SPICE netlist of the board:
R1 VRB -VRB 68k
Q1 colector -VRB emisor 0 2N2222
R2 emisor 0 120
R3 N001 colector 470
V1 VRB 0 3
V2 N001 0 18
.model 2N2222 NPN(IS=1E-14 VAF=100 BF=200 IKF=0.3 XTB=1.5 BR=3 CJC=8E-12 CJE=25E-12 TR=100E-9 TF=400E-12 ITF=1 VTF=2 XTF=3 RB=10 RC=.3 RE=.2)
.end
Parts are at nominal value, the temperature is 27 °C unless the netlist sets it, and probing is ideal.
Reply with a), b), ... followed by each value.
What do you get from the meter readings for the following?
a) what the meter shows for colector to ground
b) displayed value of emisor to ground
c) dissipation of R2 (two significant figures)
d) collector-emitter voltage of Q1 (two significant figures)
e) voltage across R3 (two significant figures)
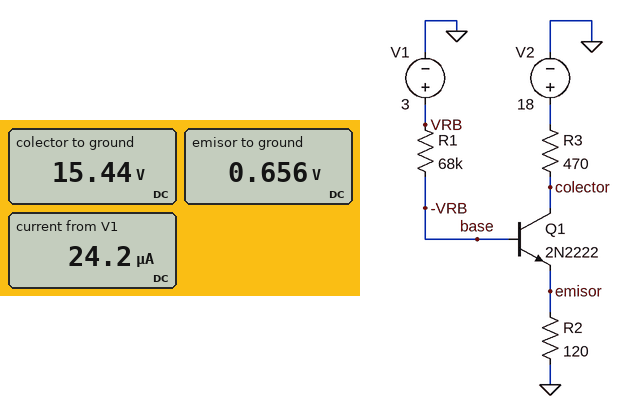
a) 15.44 V
b) 0.656 V
c) 3.6 mW
d) 15 V
e) 2.6 V
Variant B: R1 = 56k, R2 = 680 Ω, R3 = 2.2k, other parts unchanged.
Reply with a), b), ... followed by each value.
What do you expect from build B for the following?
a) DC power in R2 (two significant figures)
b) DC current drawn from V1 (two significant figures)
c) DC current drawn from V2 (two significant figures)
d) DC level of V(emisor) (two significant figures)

a) 4.2 mW
b) 11 µA
c) 2.5 mA
d) 1.7 V
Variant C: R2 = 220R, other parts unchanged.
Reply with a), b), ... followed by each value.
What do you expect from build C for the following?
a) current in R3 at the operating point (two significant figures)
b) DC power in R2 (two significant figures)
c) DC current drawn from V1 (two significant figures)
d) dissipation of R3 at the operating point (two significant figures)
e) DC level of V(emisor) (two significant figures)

a) 4.4 mA
b) 4.3 mW
c) 20 µA
d) 9.2 mW
e) 980 mV
